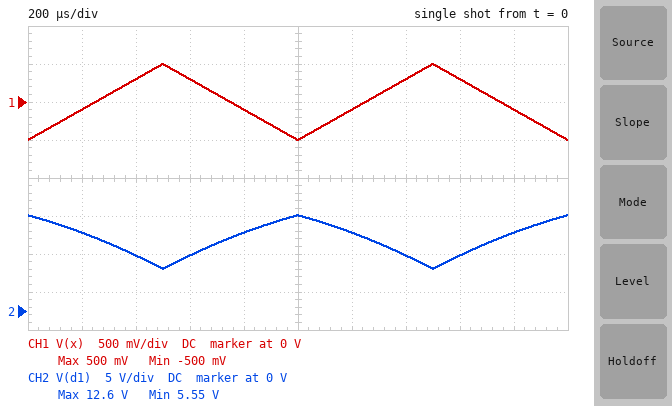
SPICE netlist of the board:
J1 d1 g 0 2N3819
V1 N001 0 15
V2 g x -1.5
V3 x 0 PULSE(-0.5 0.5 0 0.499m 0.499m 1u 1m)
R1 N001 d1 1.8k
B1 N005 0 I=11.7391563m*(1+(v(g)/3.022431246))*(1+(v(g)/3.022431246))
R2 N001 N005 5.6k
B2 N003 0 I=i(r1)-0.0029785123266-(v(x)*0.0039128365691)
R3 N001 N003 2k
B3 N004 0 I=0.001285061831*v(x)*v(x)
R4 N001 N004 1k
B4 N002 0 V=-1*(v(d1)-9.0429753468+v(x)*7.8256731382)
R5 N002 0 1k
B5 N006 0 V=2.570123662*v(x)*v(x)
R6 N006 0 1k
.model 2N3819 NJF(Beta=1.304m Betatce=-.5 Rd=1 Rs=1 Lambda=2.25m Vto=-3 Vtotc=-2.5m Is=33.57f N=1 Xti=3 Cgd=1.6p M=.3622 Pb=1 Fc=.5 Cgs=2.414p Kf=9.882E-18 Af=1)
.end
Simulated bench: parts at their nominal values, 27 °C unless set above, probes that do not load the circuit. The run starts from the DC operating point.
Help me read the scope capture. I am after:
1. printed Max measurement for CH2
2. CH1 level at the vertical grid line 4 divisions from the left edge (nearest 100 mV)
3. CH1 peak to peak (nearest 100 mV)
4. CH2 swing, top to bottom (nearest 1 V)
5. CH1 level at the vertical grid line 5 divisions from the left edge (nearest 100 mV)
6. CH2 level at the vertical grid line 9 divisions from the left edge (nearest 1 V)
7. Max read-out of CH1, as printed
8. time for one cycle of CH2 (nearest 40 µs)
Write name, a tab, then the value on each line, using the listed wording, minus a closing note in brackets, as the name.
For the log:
printed Max measurement for CH2	12.6 V
CH1 level at the vertical grid line 4 divisions from the left edge	-100 mV
CH1 peak to peak	1.0 V
CH2 swing, top to bottom	7 V
CH1 level at the vertical grid line 5 divisions from the left edge	-500 mV
CH2 level at the vertical grid line 9 divisions from the left edge	10 V
Max read-out of CH1, as printed	500 mV
time for one cycle of CH2	1.00 ms
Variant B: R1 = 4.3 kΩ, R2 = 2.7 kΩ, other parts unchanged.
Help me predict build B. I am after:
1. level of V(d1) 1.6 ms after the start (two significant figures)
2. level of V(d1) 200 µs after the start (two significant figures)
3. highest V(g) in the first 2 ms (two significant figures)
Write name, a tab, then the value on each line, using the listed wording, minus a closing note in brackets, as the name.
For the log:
level of V(d1) 1.6 ms after the start	950 mV
level of V(d1) 200 µs after the start	3.9 V
highest V(g) in the first 2 ms	-1.0 V
